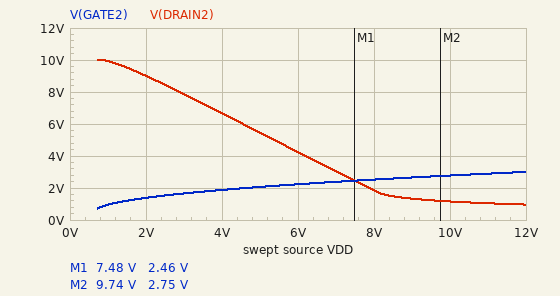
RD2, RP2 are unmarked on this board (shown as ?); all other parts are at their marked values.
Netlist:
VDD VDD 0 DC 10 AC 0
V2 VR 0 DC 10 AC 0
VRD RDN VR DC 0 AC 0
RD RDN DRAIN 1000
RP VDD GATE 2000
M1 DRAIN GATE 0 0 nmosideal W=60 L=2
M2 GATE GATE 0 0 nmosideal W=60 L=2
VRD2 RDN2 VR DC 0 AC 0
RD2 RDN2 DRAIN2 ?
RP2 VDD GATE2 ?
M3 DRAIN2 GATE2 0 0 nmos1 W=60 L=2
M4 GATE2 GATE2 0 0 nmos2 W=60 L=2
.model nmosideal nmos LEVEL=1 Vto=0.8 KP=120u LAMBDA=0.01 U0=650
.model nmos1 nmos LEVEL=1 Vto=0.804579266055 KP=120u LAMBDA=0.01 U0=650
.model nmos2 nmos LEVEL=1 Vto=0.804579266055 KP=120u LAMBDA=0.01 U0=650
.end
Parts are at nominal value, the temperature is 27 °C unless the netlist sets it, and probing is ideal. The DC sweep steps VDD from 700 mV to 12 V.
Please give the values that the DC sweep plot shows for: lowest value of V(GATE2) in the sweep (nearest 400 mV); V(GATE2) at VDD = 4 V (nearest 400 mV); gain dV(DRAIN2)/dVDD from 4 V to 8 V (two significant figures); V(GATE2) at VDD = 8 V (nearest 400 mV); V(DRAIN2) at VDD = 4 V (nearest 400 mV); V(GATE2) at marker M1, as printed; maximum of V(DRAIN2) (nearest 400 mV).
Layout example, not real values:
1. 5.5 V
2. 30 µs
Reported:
1. 800 mV
2. 2.0 V
3. -1.2 V/V
4. 2.4 V
5. 6.8 V
6. 2.46 V
7. 10.0 V
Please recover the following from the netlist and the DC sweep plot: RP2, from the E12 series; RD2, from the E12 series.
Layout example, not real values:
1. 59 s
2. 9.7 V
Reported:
1. 1 kΩ
2. 1.5 kΩ
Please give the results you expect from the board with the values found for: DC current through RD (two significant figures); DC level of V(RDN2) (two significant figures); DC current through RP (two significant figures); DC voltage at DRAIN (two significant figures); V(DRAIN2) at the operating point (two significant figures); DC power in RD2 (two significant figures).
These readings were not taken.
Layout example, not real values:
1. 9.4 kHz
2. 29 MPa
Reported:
1. 4.0 mA
2. 10 V
3. 3.9 mA
4. 6.0 V
5. 1.2 V
6. 52 mW
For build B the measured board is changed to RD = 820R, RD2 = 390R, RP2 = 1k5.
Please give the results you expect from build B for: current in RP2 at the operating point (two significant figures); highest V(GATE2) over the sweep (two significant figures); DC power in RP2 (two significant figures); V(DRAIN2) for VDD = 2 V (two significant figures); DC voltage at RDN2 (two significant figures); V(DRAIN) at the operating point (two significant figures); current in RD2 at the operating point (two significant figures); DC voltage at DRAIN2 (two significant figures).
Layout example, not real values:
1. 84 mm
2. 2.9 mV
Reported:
1. 5.0 mA
2. 2.6 V
3. 38 mW
4. 9.8 V
5. 10 V
6. 6.7 V
7. 5.3 mA
8. 7.9 V
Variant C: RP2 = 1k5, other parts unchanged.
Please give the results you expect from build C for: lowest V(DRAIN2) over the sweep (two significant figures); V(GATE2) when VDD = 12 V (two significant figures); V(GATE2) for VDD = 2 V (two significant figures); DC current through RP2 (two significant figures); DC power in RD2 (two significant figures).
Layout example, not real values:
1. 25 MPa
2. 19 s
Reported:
1. 1.4 V
2. 2.6 V
3. 1.3 V
4. 5.0 mA
5. 38 mW
